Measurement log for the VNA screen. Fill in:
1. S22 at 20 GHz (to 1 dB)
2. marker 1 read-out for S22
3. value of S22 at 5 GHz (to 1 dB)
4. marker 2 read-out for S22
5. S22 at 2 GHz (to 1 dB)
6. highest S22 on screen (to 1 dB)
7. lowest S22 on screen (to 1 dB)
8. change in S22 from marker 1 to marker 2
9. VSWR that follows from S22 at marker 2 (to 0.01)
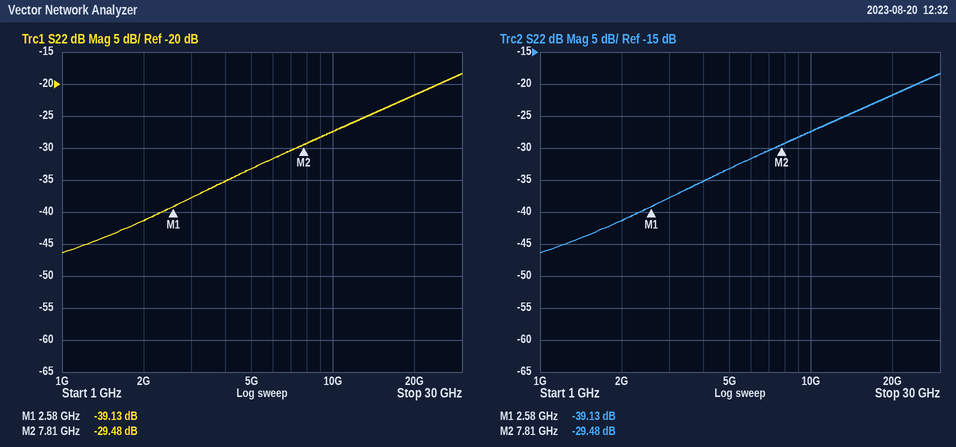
-22 dB
-39.13 dB
-33 dB
-29.48 dB
-41 dB
-18 dB
-46 dB
9.65 dB
1.07
